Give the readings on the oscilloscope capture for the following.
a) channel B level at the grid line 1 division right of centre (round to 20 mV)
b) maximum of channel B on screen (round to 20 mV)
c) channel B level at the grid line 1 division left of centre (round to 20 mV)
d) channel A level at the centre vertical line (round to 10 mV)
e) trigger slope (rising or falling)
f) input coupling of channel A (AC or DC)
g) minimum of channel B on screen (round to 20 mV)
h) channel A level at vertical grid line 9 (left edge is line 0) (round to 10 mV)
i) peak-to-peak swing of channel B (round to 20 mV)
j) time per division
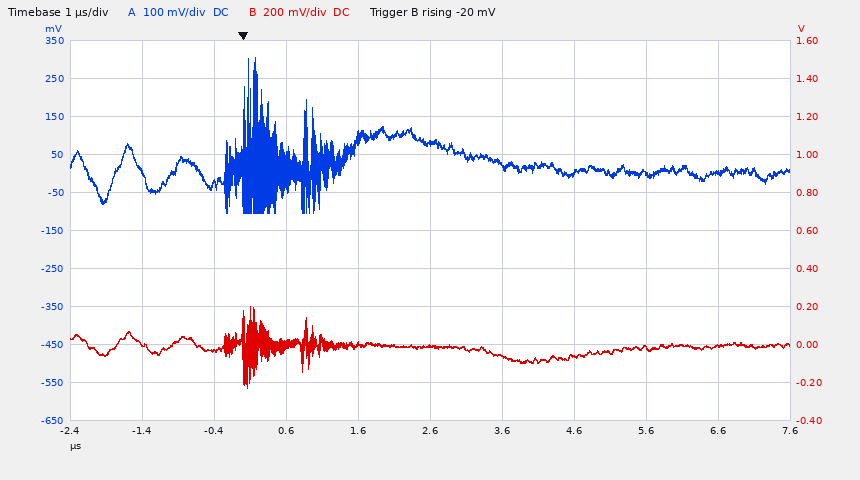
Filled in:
-60 mV
200 mV
0 mV
80 mV
rising
DC
-240 mV
0 mV
440 mV
1 µs
